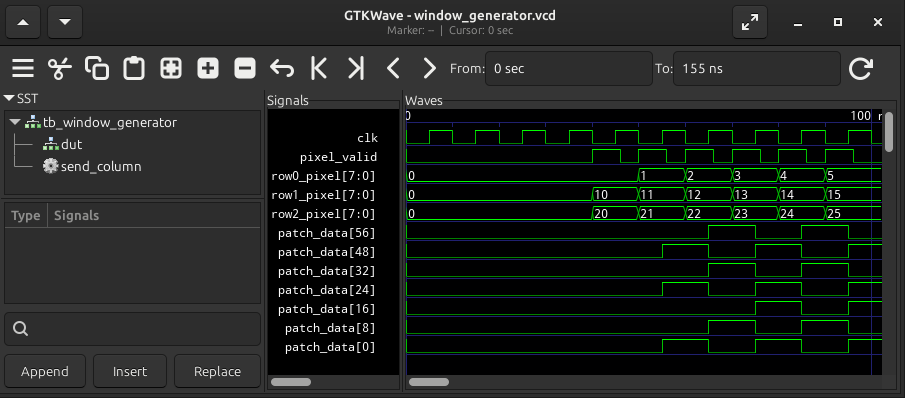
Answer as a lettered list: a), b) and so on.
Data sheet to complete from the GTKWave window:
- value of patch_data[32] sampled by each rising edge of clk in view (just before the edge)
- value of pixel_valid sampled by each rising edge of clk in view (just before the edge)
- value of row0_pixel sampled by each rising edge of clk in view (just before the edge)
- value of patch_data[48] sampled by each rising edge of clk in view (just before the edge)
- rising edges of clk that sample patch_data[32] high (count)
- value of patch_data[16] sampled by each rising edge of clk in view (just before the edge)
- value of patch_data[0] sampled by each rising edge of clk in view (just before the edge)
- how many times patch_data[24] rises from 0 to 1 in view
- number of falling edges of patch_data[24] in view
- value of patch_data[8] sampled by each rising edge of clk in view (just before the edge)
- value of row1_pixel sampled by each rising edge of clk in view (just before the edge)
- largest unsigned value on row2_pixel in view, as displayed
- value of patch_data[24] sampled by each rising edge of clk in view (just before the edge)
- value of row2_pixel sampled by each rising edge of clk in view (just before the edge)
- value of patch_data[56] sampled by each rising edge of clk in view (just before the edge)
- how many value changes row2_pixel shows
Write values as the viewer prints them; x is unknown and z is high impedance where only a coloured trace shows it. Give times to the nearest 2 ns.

a) 0 0 0 0 0 0 0 1 0 1
b) 0 0 0 0 1 1 1 1 1 1
c) 0, 0, 0, 0, 0, 1, 2, 3, 4, 5
d) 0 0 0 0 0 0 1 0 1 0
e) 2
f) 0 0 0 0 0 0 0 0 1 0
g) 0 0 0 0 0 0 1 0 1 0
h) 3
i) 2
j) 0 0 0 0 0 0 0 1 0 1
k) 0, 0, 0, 0, 10, 11, 12, 13, 14, 15
l) 25
m) 0 0 0 0 0 0 1 0 1 0
n) 0, 0, 0, 0, 20, 21, 22, 23, 24, 25
o) 0 0 0 0 0 0 0 1 0 1
p) 6
